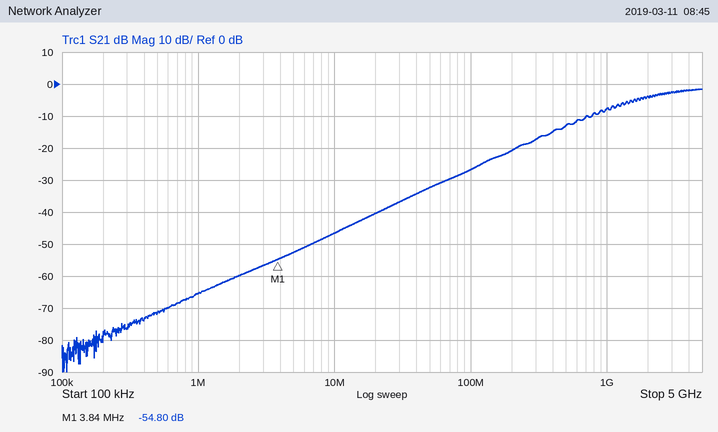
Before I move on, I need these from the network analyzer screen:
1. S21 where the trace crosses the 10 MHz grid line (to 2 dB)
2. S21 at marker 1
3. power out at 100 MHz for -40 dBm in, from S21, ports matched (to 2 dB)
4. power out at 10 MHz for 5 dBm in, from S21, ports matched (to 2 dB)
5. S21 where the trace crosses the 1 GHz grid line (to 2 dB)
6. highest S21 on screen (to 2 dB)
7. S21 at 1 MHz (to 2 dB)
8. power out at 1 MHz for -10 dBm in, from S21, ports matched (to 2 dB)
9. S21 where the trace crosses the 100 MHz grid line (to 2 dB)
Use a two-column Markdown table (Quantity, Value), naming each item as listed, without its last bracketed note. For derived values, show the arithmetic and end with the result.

| Quantity | Value |
|---|---|
| S21 where the trace crosses the 10 MHz grid line | -46 dB |
| S21 at marker 1 | -54.80 dB |
| power out at 100 MHz for -40 dBm in, from S21, ports matched | -40 dBm + (-26 dB) = -66 dBm |
| power out at 10 MHz for 5 dBm in, from S21, ports matched | 5 dBm + (-46 dB) = -42 dBm |
| S21 where the trace crosses the 1 GHz grid line | -8 dB |
| highest S21 on screen | -2 dB |
| S21 at 1 MHz | -66 dB |
| power out at 1 MHz for -10 dBm in, from S21, ports matched | -10 dBm + (-66 dB) = -76 dBm |
| S21 where the trace crosses the 100 MHz grid line | -26 dB |
